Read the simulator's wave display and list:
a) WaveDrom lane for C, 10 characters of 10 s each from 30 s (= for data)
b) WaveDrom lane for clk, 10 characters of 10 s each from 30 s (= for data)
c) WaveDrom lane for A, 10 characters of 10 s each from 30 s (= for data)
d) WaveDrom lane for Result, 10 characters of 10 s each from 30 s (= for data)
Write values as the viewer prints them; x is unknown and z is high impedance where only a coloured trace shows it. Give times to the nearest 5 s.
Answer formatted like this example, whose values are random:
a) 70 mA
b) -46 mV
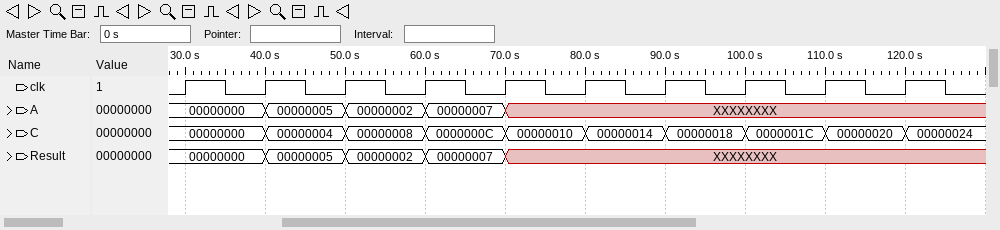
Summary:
a) {name: 'C', wave: '==========', data: '00000000 00000004 00000008 0000000C 00000010 00000014 00000018 0000001C 00000020 00000024'}
b) {name: 'clk', wave: 'p.........'}
c) {name: 'A', wave: '====x.....', data: '00000000 00000005 00000002 00000007'}
d) {name: 'Result', wave: '====x.....', data: '00000000 00000005 00000002 00000007'}
